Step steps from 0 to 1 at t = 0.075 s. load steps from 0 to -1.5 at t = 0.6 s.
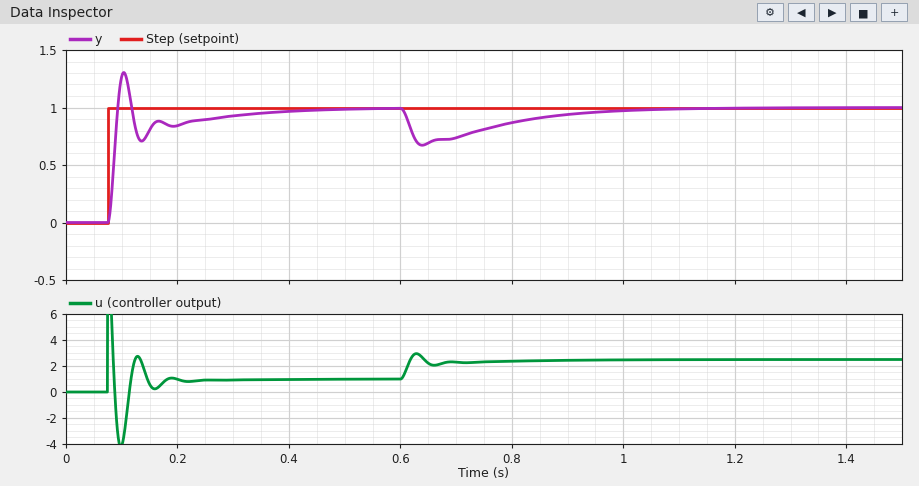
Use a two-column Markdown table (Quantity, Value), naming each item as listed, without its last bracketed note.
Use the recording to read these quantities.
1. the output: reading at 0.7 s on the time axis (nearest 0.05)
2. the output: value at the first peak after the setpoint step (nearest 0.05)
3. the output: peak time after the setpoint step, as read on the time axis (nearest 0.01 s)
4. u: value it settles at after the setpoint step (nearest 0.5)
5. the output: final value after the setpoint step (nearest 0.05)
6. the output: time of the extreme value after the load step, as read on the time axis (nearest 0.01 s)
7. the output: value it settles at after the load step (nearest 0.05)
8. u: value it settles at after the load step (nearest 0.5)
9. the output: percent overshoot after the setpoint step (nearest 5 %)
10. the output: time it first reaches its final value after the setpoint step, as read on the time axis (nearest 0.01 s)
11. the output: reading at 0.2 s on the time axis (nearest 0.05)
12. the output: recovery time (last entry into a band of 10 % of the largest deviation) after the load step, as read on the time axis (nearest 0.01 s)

| Quantity | Value |
|---|---|
| the output: reading at 0.7 s on the time axis | 0.75 |
| the output: value at the first peak after the setpoint step | 1.30 |
| the output: peak time after the setpoint step, as read on the time axis | 0.10 s |
| u: value it settles at after the setpoint step | 1.0 |
| the output: final value after the setpoint step | 1.00 |
| the output: time of the extreme value after the load step, as read on the time axis | 0.64 s |
| the output: value it settles at after the load step | 1.00 |
| u: value it settles at after the load step | 2.5 |
| the output: percent overshoot after the setpoint step | 30 % |
| the output: time it first reaches its final value after the setpoint step, as read on the time axis | 0.09 s |
| the output: reading at 0.2 s on the time axis | 0.85 |
| the output: recovery time (last entry into a band of 10 % of the largest deviation) after the load step, as read on the time axis | 0.98 s |
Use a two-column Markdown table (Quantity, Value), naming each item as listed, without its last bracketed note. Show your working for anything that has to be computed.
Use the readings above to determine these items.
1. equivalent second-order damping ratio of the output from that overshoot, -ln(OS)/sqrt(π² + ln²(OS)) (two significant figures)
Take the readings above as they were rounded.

| Quantity | Value |
|---|---|
| equivalent second-order damping ratio of the output from that overshoot, -ln(OS)/sqrt(π² + ln²(OS)) | ln(0.3) = -1.204; 1.204 / sqrt(9.870 + 1.450) = 0.36 |
